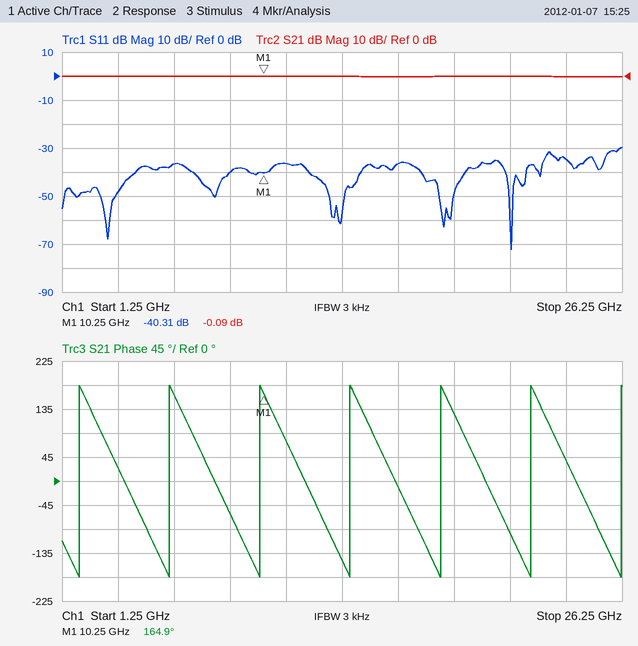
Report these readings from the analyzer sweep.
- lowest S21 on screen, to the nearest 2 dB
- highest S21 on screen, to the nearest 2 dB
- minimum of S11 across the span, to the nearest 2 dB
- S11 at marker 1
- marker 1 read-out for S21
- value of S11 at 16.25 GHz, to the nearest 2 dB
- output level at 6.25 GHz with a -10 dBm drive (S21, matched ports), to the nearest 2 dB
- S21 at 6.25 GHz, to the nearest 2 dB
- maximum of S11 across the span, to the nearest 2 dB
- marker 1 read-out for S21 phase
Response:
0 dB
0 dB
-72 dB
-40.31 dB
-0.09 dB
-36 dB
-10 dBm
0 dB
-30 dB
164.9°
